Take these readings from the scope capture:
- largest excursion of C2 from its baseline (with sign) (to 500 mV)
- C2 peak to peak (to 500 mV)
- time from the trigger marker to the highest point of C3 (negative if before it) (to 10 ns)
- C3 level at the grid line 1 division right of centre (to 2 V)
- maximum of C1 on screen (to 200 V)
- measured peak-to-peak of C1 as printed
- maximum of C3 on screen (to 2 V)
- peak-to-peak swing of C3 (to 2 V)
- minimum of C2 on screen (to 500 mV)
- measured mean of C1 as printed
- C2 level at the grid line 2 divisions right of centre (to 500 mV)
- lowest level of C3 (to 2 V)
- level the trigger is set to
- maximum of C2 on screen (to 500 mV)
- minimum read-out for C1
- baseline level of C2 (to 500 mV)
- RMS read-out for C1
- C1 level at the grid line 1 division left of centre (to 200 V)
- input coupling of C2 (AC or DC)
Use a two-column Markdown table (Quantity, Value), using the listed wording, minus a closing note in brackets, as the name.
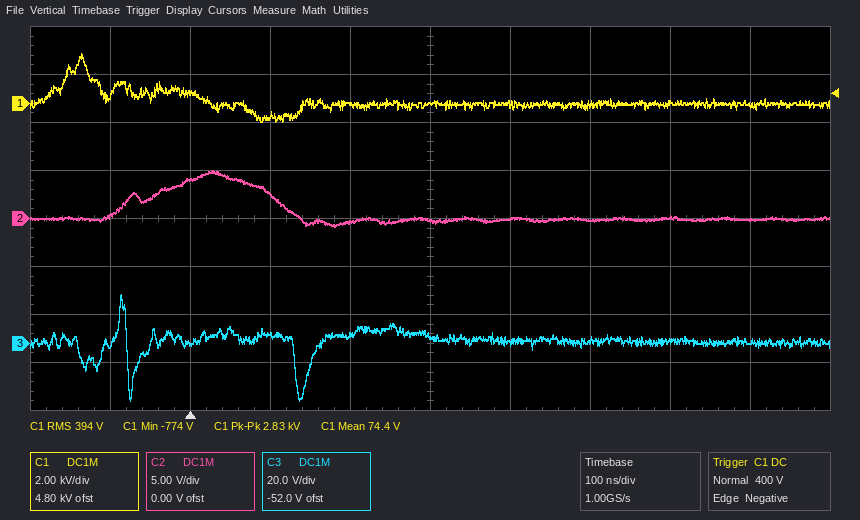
| Quantity | Value |
|---|---|
| largest excursion of C2 from its baseline (with sign) | +5.0 V |
| C2 peak to peak | 6.0 V |
| time from the trigger marker to the highest point of C3 (negative if before it) | -90 ns |
| C3 level at the grid line 1 division right of centre | 0 V |
| maximum of C1 on screen | 2.0 kV |
| measured peak-to-peak of C1 as printed | 2.83 kV |
| maximum of C3 on screen | 20 V |
| peak-to-peak swing of C3 | 44 V |
| minimum of C2 on screen | -1.0 V |
| measured mean of C1 as printed | 74.4 V |
| C2 level at the grid line 2 divisions right of centre | 0.0 V |
| lowest level of C3 | -24 V |
| level the trigger is set to | 400 V |
| maximum of C2 on screen | 5.0 V |
| minimum read-out for C1 | -774 V |
| baseline level of C2 | 0.0 V |
| RMS read-out for C1 | 394 V |
| C1 level at the grid line 1 division left of centre | 0.0 kV |
| input coupling of C2 | DC |
